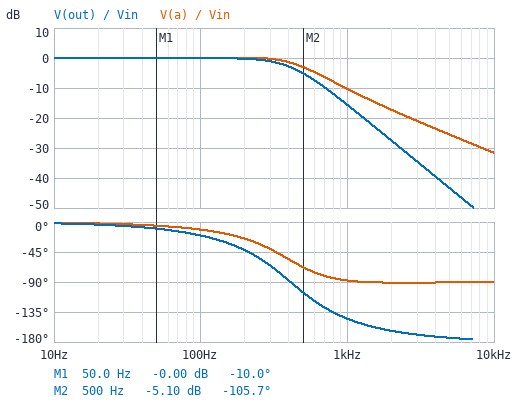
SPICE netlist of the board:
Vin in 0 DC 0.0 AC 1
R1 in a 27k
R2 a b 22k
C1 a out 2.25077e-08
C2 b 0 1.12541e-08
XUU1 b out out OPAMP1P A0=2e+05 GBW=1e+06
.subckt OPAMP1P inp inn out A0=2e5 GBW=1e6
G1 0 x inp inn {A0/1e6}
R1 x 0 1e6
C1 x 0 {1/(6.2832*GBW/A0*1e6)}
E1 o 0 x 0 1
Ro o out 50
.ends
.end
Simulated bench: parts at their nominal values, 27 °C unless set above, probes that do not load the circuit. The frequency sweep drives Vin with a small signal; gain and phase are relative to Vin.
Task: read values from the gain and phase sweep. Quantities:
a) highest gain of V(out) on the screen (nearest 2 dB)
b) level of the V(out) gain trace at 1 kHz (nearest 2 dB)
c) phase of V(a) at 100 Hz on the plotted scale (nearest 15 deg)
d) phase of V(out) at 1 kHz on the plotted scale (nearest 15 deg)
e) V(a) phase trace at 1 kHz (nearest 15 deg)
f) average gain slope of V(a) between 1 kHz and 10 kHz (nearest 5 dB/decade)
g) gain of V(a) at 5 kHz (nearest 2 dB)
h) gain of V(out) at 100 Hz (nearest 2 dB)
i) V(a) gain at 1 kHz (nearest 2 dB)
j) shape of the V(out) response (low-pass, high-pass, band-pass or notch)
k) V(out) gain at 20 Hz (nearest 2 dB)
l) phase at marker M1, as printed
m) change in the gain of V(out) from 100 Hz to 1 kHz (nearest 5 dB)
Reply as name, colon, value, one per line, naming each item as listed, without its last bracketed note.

highest gain of V(out) on the screen: 0 dB
level of the V(out) gain trace at 1 kHz: -16 dB
phase of V(a) at 100 Hz on the plotted scale: -15 deg
phase of V(out) at 1 kHz on the plotted scale: -150 deg
V(a) phase trace at 1 kHz: -90 deg
average gain slope of V(a) between 1 kHz and 10 kHz: -20 dB/decade
gain of V(a) at 5 kHz: -26 dB
gain of V(out) at 100 Hz: 0 dB
V(a) gain at 1 kHz: -10 dB
shape of the V(out) response: low-pass
V(out) gain at 20 Hz: 0 dB
phase at marker M1, as printed: -10.0 deg
change in the gain of V(out) from 100 Hz to 1 kHz: -15 dB
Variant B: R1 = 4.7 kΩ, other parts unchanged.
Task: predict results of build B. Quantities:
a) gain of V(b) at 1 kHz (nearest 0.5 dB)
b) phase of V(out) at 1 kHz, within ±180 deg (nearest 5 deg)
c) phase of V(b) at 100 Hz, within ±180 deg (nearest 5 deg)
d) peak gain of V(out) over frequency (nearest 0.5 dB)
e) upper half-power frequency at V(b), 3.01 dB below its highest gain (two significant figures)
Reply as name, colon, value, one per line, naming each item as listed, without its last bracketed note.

gain of V(b) at 1 kHz: -5.5 dB
phase of V(out) at 1 kHz, within ±180 deg: -90 deg
phase of V(b) at 100 Hz, within ±180 deg: -10 deg
peak gain of V(out) over frequency: 0 dB
upper half-power frequency at V(b), 3.01 dB below its highest gain: 700 Hz
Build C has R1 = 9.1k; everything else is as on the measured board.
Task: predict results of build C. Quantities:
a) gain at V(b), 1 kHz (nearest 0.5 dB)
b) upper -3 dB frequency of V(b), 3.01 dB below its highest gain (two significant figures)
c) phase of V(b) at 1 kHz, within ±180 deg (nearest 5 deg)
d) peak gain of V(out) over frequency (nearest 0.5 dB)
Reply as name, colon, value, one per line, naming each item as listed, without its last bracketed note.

gain at V(b), 1 kHz: -7.5 dB
upper -3 dB frequency of V(b), 3.01 dB below its highest gain: 640 Hz
phase of V(b) at 1 kHz, within ±180 deg: -115 deg
peak gain of V(out) over frequency: 0 dB
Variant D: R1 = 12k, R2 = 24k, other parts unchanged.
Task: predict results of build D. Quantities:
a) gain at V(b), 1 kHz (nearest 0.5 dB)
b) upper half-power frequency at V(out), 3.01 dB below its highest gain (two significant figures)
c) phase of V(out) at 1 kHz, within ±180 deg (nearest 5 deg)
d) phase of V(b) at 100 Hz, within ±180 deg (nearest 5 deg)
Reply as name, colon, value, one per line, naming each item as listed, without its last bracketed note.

gain at V(b), 1 kHz: -10.0 dB
upper half-power frequency at V(out), 3.01 dB below its highest gain: 550 Hz
phase of V(out) at 1 kHz, within ±180 deg: -125 deg
phase of V(b) at 100 Hz, within ±180 deg: -15 deg
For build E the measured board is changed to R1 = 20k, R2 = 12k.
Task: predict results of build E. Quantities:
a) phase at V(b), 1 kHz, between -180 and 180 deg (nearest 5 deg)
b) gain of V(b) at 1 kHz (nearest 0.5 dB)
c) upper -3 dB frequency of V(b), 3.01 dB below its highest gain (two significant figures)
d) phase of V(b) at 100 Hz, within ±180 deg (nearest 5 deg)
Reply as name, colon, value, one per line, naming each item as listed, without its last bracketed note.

phase at V(b), 1 kHz, between -180 and 180 deg: -120 deg
gain of V(b) at 1 kHz: -8.5 dB
upper -3 dB frequency of V(b), 3.01 dB below its highest gain: 620 Hz
phase of V(b) at 100 Hz, within ±180 deg: -15 deg
